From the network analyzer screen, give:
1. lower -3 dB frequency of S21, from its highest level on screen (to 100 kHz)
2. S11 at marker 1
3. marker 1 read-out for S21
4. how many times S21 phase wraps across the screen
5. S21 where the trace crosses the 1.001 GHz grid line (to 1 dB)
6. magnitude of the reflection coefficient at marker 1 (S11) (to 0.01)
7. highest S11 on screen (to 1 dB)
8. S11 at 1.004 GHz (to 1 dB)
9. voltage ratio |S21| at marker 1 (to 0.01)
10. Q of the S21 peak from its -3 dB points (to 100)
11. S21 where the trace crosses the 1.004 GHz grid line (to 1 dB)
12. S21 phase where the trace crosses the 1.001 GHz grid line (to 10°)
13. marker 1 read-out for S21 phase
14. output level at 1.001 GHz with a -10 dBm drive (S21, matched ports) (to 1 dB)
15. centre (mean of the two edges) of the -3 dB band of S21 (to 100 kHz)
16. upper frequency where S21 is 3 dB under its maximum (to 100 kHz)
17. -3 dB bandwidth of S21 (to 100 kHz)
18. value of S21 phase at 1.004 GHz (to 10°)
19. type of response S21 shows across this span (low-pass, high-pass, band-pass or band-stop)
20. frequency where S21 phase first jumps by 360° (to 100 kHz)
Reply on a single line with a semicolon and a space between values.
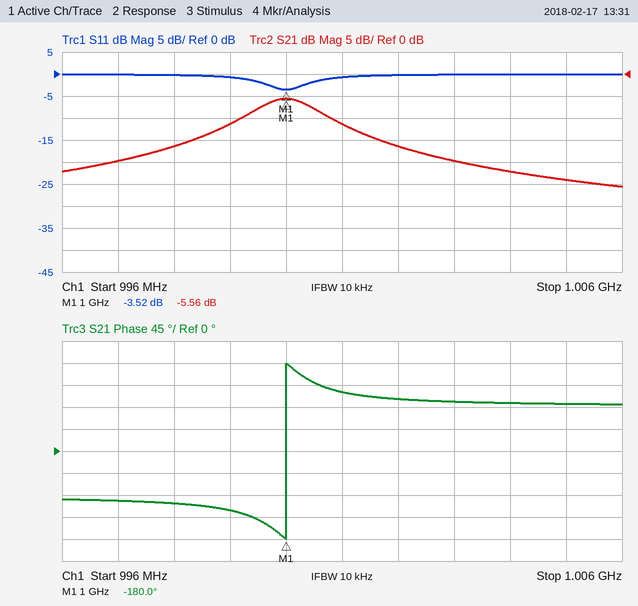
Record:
999.4 MHz; -3.52 dB; -5.56 dB; 1; -11 dB; 0.67; 0 dB; 0 dB; 0.53; 800; -22 dB; 120°; -180.0°; -21 dBm; 1.0000 GHz; 1.0006 GHz; 1.2 MHz; 100°; band-pass; 1.0000 GHz
